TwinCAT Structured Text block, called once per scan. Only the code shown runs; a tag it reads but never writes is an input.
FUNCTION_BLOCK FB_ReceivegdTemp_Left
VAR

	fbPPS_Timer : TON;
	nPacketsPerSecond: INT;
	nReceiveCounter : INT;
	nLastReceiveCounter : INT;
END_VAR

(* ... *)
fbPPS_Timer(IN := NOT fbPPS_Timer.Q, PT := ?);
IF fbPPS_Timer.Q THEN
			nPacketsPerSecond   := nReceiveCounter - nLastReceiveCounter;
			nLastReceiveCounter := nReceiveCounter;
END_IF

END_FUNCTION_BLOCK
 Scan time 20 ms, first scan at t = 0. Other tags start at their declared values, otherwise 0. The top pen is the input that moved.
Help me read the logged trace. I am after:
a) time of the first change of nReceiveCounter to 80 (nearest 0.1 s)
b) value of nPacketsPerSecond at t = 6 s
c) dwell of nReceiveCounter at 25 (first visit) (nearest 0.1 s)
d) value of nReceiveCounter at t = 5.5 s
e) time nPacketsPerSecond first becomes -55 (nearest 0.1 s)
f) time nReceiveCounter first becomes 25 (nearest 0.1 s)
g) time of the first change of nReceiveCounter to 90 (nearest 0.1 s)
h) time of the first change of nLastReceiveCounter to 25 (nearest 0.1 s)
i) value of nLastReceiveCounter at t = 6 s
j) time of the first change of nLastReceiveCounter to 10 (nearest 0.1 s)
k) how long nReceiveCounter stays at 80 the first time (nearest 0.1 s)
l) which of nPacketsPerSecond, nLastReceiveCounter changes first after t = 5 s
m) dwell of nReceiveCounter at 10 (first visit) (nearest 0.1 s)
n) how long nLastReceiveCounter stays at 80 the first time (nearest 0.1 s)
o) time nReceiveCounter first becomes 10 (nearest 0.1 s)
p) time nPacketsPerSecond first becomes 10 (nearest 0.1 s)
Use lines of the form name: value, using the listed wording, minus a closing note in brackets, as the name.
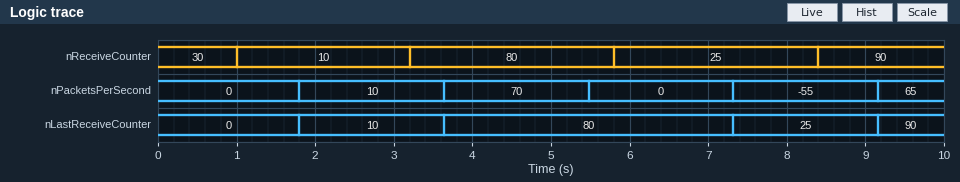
time of the first change of nReceiveCounter to 80: 3.2 s
value of nPacketsPerSecond at t = 6 s: 0
dwell of nReceiveCounter at 25 (first visit): 2.6 s
value of nReceiveCounter at t = 5.5 s: 80
time nPacketsPerSecond first becomes -55: 7.3 s
time nReceiveCounter first becomes 25: 5.8 s
time of the first change of nReceiveCounter to 90: 8.4 s
time of the first change of nLastReceiveCounter to 25: 7.3 s
value of nLastReceiveCounter at t = 6 s: 80
time of the first change of nLastReceiveCounter to 10: 1.8 s
how long nReceiveCounter stays at 80 the first time: 2.6 s
which of nPacketsPerSecond, nLastReceiveCounter changes first after t = 5 s: nPacketsPerSecond
dwell of nReceiveCounter at 10 (first visit): 2.2 s
how long nLastReceiveCounter stays at 80 the first time: 3.7 s
time nReceiveCounter first becomes 10: 1.0 s
time nPacketsPerSecond first becomes 10: 1.8 s
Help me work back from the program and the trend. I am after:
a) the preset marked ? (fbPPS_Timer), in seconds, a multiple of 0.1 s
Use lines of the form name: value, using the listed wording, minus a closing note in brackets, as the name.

the preset marked ? (fbPPS_Timer), in seconds, a multiple of 0.1 s: 1.8 s
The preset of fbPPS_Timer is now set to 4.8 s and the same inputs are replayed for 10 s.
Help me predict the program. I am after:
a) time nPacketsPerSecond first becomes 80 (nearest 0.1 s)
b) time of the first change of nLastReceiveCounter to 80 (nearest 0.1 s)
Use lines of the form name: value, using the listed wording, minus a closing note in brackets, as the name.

time nPacketsPerSecond first becomes 80: 4.8 s
time of the first change of nLastReceiveCounter to 80: 4.8 s
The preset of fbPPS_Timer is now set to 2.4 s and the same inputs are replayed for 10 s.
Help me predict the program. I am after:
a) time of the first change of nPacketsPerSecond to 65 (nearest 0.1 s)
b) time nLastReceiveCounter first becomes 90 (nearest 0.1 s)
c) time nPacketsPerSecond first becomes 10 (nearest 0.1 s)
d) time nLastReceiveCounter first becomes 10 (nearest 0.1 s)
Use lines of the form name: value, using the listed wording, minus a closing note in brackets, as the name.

time of the first change of nPacketsPerSecond to 65: 9.7 s
time nLastReceiveCounter first becomes 90: 9.7 s
time nPacketsPerSecond first becomes 10: 2.4 s
time nLastReceiveCounter first becomes 10: 2.4 s
